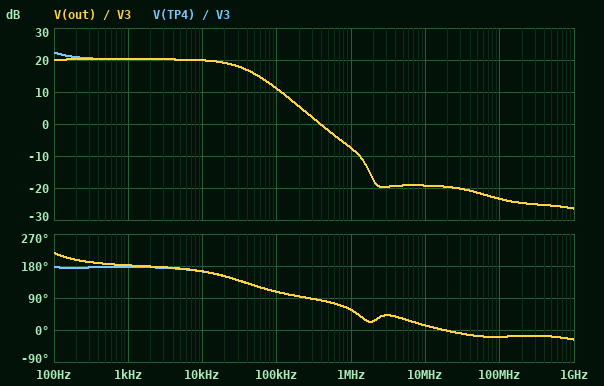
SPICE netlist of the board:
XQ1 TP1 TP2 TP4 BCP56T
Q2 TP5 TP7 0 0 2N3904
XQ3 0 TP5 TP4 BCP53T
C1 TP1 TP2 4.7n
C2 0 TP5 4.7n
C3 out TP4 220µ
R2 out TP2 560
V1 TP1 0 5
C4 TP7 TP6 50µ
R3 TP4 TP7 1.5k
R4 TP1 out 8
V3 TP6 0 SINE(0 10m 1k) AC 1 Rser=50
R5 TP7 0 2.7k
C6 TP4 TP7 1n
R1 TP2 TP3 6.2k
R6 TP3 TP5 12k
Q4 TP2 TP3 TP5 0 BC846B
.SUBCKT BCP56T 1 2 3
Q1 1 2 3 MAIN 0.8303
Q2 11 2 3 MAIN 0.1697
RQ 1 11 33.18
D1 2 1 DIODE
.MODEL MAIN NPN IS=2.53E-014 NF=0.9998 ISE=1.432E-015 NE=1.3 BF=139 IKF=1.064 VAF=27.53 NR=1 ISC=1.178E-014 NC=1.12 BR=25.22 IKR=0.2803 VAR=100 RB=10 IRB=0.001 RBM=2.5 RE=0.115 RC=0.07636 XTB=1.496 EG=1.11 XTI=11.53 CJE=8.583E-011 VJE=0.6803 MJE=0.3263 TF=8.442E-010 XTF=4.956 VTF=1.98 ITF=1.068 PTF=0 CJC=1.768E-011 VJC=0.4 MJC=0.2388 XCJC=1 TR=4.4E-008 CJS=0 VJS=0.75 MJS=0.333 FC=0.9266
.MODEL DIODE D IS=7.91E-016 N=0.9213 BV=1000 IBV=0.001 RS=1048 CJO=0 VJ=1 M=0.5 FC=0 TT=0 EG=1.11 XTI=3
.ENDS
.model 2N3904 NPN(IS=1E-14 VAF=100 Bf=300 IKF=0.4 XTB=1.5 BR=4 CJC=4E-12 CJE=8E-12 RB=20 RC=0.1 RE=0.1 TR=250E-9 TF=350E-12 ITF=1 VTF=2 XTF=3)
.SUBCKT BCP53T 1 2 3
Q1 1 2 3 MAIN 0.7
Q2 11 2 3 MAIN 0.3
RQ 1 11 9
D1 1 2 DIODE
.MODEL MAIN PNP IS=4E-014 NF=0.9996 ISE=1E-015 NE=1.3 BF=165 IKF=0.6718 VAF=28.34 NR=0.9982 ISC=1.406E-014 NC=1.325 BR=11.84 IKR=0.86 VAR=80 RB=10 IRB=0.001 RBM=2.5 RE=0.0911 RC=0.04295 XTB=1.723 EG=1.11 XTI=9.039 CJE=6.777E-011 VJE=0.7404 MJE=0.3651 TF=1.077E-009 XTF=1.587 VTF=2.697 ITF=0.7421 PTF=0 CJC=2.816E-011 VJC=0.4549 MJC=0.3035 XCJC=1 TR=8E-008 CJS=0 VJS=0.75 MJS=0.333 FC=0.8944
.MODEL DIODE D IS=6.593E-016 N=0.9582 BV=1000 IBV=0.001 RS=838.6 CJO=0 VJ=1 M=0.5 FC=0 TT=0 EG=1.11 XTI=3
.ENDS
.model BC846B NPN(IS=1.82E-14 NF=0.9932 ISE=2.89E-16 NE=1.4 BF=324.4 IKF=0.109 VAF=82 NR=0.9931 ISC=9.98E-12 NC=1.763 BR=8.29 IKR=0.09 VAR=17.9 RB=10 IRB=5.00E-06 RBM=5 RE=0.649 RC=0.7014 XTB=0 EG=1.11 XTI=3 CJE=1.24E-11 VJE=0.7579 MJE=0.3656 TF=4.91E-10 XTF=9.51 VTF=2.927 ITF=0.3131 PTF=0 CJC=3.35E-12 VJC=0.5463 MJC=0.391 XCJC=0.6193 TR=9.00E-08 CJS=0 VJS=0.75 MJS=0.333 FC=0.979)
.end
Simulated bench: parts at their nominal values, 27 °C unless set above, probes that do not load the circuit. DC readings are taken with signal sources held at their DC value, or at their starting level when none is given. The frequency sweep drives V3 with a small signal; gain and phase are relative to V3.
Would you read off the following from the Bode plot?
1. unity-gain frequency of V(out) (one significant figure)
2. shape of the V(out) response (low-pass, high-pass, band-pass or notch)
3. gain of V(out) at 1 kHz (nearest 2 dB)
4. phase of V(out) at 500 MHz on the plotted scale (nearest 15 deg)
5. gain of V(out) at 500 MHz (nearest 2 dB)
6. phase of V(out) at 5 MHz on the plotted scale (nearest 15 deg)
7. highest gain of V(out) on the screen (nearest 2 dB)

400 kHz
low-pass
20 dB
-15 deg
-26 dB
30 deg
20 dB
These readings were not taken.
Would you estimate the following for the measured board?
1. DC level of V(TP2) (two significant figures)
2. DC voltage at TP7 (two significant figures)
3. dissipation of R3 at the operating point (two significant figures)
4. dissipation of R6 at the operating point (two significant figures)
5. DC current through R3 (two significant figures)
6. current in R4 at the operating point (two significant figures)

1.7 V
700 mV
120 µW
39 µW
280 µA
5.8 mA
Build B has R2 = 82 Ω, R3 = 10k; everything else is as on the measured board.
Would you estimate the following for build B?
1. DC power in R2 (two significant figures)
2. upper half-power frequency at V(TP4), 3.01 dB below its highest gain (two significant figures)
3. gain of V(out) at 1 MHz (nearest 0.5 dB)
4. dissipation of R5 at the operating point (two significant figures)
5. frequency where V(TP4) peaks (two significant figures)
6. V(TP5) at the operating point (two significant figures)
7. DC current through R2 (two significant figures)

5.7 mW
120 Hz
1.0 dB
190 µW
26 Hz
3.0 V
8.3 mA
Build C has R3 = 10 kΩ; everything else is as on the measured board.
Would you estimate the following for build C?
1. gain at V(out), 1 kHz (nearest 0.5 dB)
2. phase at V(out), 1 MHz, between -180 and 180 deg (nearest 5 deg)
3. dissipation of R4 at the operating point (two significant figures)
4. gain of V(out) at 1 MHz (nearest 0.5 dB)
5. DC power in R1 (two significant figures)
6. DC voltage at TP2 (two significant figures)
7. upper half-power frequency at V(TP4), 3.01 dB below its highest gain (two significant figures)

11.5 dB
40 deg
34 µW
-17.5 dB
23 µW
3.8 V
18 Hz
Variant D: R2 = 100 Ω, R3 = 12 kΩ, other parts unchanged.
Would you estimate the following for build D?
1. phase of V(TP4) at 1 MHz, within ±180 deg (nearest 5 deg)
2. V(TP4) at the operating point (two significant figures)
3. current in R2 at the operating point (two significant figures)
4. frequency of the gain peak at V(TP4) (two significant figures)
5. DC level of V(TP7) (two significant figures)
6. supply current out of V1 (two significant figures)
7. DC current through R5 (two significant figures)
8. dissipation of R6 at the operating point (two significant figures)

50 deg
3.9 V
4.3 mA
8.0 Hz
690 mV
4.6 mA
260 µA
38 µW
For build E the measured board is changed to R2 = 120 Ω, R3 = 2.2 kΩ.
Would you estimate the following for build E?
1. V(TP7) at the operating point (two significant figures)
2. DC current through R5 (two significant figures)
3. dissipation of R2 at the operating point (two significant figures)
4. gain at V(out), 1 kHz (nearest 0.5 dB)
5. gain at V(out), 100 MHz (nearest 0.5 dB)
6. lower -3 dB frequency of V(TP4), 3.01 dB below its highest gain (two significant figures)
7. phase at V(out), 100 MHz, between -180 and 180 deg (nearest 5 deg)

740 mV
270 µA
54 mW
32.0 dB
-31.0 dB
100 Hz
35 deg
